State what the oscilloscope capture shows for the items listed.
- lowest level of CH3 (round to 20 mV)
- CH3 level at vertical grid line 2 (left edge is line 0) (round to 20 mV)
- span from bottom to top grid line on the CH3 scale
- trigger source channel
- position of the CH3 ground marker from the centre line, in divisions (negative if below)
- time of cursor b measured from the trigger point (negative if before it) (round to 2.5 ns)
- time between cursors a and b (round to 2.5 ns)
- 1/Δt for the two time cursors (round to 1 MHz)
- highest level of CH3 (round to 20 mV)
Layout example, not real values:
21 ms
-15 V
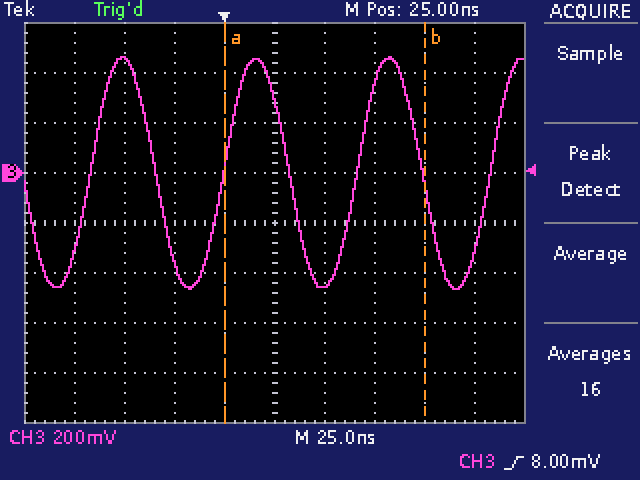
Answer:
-460 mV
460 mV
1.6 V
CH3
+1.0 div
+100.0 ns
100.0 ns
10 MHz
460 mV
